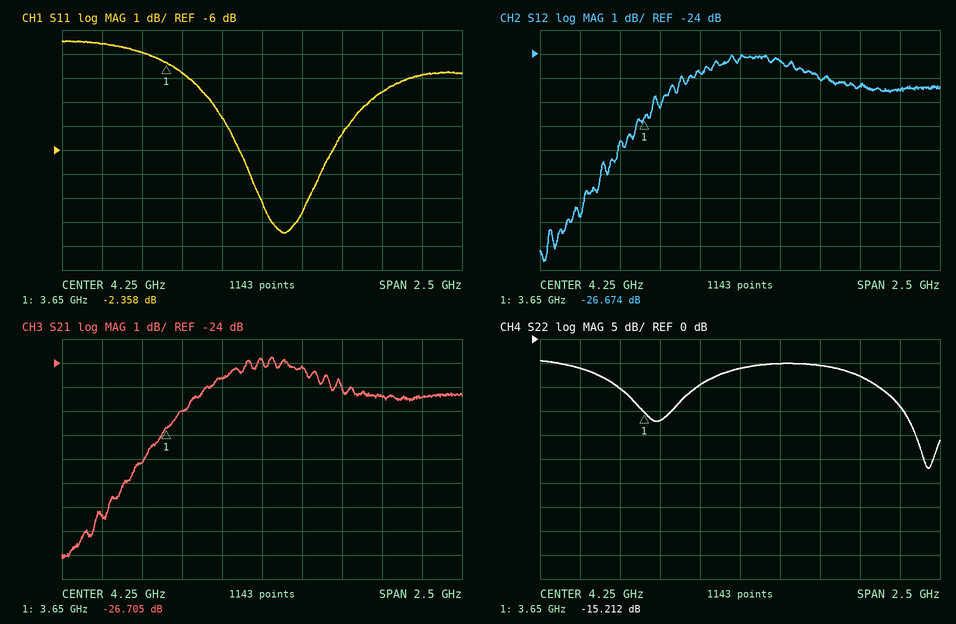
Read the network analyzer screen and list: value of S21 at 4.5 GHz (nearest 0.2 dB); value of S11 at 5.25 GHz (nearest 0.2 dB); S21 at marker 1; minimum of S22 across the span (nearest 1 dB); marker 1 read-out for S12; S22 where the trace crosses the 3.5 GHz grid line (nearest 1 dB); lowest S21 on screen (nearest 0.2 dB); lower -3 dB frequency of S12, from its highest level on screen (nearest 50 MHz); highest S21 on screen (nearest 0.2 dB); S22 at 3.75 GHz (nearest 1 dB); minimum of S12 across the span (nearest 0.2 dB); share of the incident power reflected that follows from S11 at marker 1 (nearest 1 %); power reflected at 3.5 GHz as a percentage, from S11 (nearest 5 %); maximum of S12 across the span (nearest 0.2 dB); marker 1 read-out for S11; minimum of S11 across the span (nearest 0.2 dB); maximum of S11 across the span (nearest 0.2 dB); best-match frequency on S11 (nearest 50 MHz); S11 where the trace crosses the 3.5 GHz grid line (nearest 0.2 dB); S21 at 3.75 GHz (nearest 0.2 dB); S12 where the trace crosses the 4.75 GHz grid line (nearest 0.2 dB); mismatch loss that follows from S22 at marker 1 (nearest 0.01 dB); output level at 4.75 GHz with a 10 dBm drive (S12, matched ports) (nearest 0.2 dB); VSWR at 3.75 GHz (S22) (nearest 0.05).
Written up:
-24.2 dB
-2.8 dB
-26.705 dB
-27 dB
-26.674 dB
-10 dB
-32.2 dB
3.60 GHz
-23.8 dB
-17 dB
-32.6 dB
58 %
65 %
-24.0 dB
-2.358 dB
-9.4 dB
-1.4 dB
4.40 GHz
-2.0 dB
-26.0 dB
-25.0 dB
0.13 dB
-15.0 dBm
1.35
